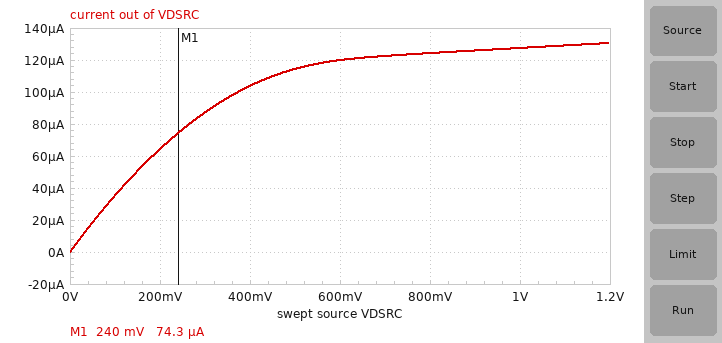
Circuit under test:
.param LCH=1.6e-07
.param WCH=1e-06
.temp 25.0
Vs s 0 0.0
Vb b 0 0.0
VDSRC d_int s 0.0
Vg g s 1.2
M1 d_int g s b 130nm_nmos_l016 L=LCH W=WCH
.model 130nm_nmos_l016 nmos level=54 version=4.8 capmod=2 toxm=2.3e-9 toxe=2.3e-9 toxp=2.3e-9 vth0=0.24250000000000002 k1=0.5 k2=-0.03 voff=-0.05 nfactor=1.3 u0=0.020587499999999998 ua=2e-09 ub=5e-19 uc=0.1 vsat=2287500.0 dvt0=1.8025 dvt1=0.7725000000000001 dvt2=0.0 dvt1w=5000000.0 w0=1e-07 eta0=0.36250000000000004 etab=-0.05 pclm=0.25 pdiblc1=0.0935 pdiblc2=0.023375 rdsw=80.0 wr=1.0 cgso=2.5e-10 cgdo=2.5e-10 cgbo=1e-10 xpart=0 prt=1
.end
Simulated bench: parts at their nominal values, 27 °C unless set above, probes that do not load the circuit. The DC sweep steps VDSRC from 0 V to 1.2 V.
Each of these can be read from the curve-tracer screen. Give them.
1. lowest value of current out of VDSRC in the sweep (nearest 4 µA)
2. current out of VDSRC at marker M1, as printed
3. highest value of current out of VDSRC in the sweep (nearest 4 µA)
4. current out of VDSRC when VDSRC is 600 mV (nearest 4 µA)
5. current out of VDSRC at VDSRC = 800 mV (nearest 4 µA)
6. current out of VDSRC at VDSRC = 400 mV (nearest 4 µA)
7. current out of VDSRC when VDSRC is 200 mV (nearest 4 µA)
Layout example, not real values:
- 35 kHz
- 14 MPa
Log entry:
- 0 A
- 74.3 µA
- 132 µA
- 120 µA
- 124 µA
- 104 µA
- 64 µA
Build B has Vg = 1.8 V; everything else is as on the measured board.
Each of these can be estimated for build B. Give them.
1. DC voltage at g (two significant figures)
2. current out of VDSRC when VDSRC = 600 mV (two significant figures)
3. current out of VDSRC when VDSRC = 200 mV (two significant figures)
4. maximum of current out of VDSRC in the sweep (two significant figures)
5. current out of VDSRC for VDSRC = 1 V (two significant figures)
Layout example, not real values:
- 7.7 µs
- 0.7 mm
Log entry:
- 1.8 V
- 270 µA
- 110 µA
- 360 µA
- 350 µA
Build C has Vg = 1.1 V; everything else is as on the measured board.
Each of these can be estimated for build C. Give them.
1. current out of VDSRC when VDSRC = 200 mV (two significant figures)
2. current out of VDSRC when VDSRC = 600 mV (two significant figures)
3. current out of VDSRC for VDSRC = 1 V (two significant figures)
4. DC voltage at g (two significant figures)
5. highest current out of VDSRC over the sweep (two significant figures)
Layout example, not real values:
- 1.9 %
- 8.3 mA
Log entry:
- 54 µA
- 91 µA
- 97 µA
- 1.1 V
- 100 µA
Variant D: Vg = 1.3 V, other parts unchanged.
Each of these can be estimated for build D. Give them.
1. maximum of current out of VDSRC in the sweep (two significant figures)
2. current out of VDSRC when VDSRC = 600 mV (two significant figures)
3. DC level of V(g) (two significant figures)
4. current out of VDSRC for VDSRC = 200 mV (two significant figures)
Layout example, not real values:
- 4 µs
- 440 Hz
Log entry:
- 160 µA
- 150 µA
- 1.3 V
- 74 µA
